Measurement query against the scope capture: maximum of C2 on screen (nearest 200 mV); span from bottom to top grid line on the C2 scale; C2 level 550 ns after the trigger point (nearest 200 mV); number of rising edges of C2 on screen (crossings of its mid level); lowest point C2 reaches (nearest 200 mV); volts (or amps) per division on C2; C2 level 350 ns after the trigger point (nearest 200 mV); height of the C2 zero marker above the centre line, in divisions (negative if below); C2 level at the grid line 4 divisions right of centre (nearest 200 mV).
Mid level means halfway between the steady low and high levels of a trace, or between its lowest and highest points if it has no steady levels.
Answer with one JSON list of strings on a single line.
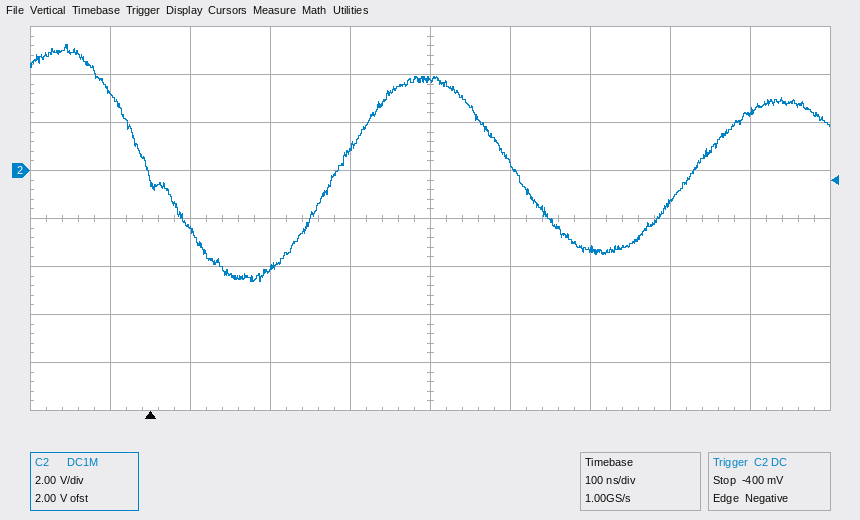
["5.2 V", "16 V", "-3.2 V", "2", "-4.6 V", "2 V", "3.8 V", "+1.0 div", "2.4 V"]
